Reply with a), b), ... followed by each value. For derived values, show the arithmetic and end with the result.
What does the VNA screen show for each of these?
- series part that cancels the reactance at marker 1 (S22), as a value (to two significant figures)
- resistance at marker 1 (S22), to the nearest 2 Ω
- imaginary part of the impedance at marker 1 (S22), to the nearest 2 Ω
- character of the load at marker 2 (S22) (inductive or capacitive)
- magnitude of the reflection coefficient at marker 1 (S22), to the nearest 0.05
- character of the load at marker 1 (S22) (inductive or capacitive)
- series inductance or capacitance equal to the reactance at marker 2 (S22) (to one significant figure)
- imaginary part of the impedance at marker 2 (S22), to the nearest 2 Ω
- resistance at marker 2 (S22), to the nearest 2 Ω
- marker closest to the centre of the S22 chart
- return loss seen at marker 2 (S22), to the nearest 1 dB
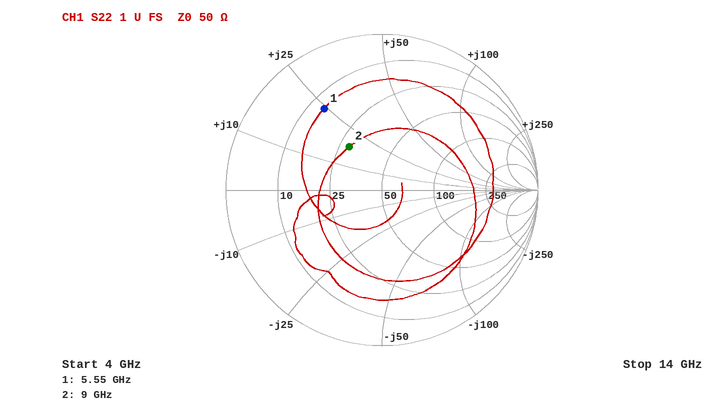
a) C = 1/(2π × 5.55 GHz × 24 Ω) ≈ 1.2 pF
b) 14 Ω
c) +24 Ω
d) inductive
e) 0.65
f) inductive
g) L = 18 Ω/(2π × 9 GHz) ≈ 318 pH, so 300 pH to one significant figure
h) +18 Ω
i) 28 Ω
j) marker 2
k) 9 dB
